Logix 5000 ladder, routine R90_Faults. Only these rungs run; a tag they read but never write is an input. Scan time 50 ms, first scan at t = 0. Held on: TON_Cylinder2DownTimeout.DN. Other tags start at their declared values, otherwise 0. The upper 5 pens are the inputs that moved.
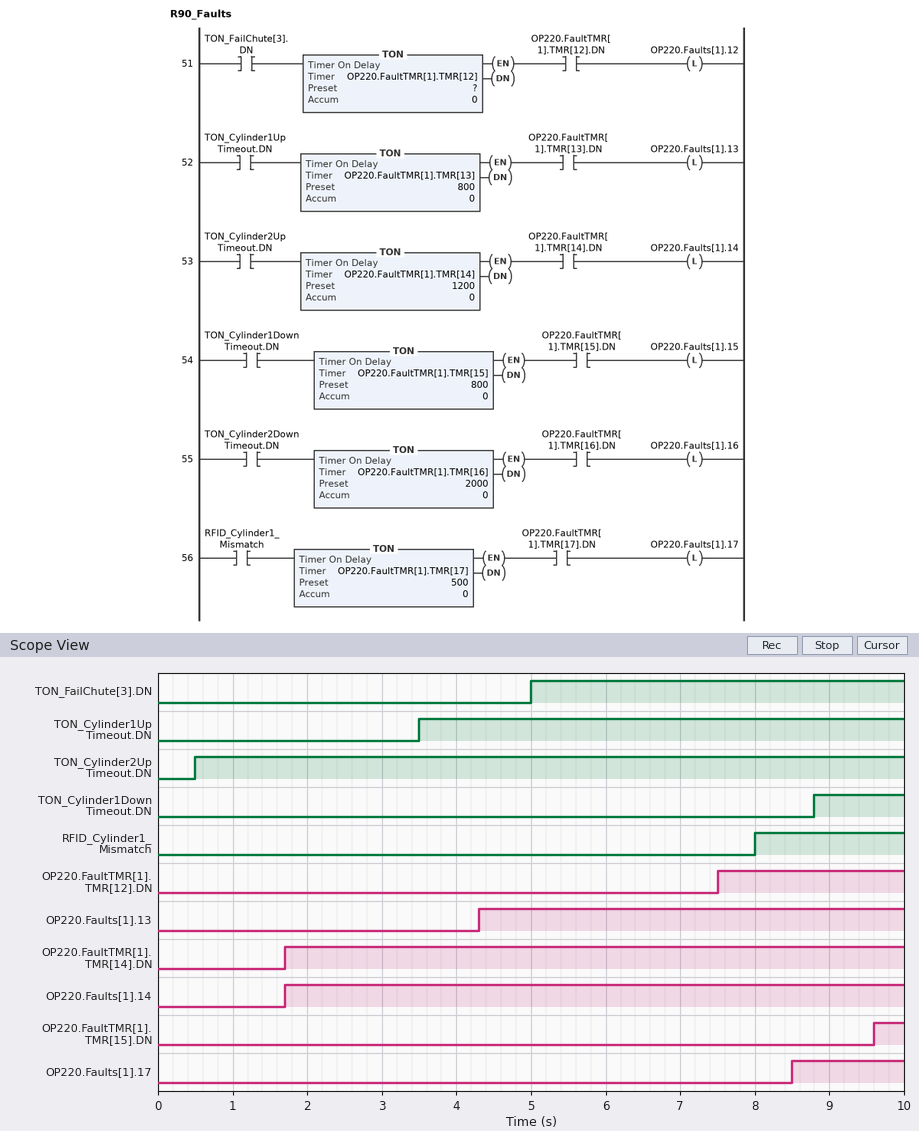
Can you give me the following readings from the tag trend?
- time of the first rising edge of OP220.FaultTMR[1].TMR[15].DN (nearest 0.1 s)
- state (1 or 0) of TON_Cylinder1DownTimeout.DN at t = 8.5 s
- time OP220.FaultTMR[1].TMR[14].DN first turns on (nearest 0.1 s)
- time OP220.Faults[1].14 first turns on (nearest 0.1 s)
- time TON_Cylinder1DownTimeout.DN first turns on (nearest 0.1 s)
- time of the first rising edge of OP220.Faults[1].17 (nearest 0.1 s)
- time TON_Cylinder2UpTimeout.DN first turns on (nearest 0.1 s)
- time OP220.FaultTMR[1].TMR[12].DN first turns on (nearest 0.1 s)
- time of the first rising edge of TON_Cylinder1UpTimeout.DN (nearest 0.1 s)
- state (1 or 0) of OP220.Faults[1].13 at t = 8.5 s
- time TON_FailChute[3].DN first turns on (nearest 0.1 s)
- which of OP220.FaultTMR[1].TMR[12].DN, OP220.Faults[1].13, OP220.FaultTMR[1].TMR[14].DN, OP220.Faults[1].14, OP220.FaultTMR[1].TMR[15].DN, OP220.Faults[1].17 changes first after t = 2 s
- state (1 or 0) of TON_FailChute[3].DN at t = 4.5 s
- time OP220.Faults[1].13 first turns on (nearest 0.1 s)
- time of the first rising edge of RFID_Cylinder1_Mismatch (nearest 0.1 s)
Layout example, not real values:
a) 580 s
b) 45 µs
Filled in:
a) 9.6 s
b) 0
c) 1.7 s
d) 1.7 s
e) 8.8 s
f) 8.5 s
g) 0.5 s
h) 7.5 s
i) 3.5 s
j) 1
k) 5.0 s
l) OP220.Faults[1].13
m) 0
n) 4.3 s
o) 8.0 s
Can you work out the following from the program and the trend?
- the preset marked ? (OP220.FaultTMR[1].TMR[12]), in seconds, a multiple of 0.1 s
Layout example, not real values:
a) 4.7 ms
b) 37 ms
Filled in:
a) 2.5 s
